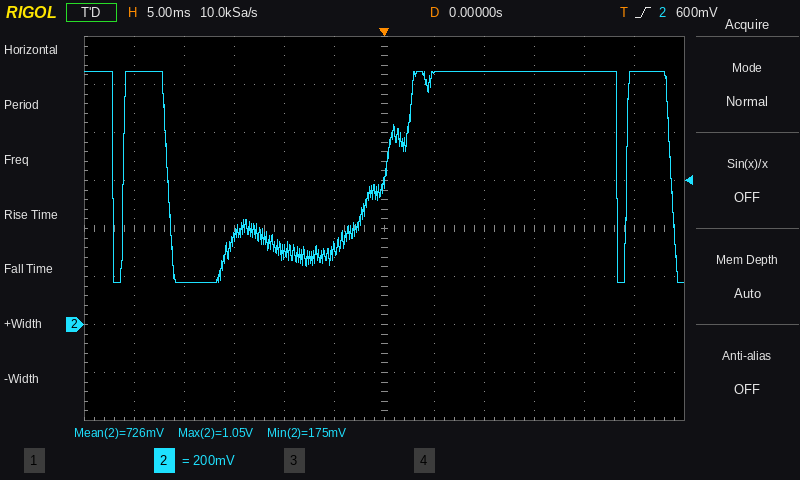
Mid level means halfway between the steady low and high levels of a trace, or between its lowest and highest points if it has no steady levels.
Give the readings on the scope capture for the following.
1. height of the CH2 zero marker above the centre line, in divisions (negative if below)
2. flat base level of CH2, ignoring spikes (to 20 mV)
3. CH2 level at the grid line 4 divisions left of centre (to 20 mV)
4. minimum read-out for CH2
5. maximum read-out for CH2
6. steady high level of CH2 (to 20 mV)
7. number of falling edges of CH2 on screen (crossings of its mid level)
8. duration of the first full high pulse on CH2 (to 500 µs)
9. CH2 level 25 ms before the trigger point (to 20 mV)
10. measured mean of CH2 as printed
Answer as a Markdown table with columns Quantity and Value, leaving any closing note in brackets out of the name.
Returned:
| Quantity | Value |
|---|---|
| height of the CH2 zero marker above the centre line, in divisions | -2.0 div |
| flat base level of CH2, ignoring spikes | 180 mV |
| CH2 level at the grid line 4 divisions left of centre | 180 mV |
| minimum read-out for CH2 | 175 mV |
| maximum read-out for CH2 | 1.05 V |
| steady high level of CH2 | 1.06 V |
| number of falling edges of CH2 on screen | 4 |
| duration of the first full high pulse on CH2 | 4.5 ms |
| CH2 level 25 ms before the trigger point | 1.06 V |
| measured mean of CH2 as printed | 726 mV |
